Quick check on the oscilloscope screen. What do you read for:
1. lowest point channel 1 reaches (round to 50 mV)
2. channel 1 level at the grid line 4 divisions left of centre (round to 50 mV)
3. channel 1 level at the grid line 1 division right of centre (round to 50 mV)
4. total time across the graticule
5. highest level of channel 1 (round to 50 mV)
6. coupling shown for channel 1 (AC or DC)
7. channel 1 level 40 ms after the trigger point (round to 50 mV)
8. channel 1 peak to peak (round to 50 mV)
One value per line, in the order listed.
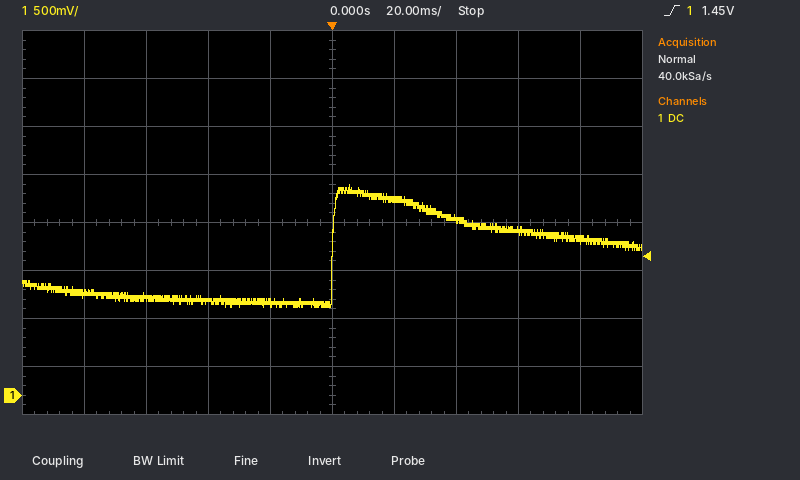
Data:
900 mV
1.05 V
2.05 V
200 ms
2.20 V
DC
1.85 V
1.30 V
